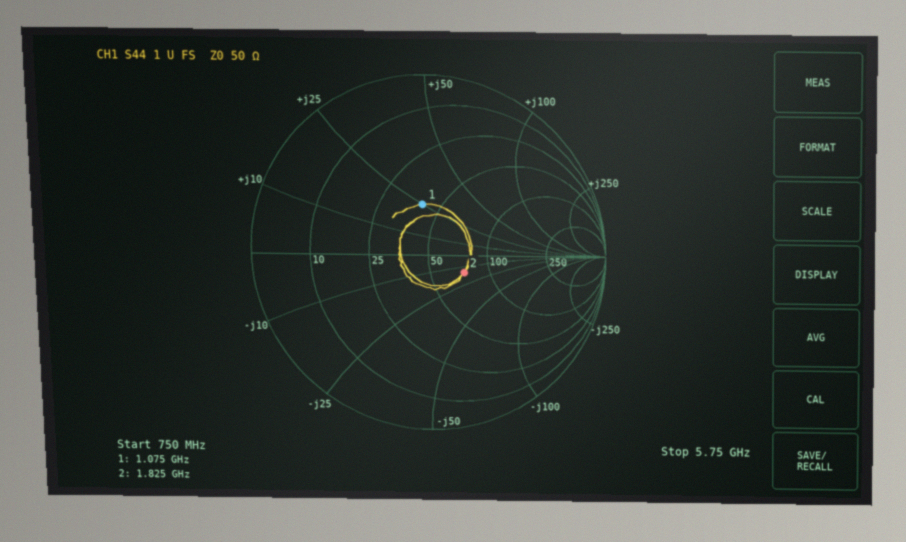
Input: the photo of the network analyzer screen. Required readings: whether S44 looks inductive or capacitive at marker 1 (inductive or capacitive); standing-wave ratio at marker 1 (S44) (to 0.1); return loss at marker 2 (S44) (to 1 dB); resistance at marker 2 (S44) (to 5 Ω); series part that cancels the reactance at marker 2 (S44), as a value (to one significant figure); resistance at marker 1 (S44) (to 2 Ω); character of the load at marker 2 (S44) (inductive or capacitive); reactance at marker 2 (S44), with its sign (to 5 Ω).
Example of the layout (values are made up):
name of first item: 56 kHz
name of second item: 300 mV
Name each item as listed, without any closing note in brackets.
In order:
whether S44 looks inductive or capacitive at marker 1: inductive
standing-wave ratio at marker 1 (S44): 1.8
return loss at marker 2 (S44): 13 dB
resistance at marker 2 (S44): 75 Ω
series part that cancels the reactance at marker 2 (S44), as a value: 1 nH
resistance at marker 1 (S44): 40 Ω
character of the load at marker 2 (S44): capacitive
reactance at marker 2 (S44), with its sign: -15 Ω
